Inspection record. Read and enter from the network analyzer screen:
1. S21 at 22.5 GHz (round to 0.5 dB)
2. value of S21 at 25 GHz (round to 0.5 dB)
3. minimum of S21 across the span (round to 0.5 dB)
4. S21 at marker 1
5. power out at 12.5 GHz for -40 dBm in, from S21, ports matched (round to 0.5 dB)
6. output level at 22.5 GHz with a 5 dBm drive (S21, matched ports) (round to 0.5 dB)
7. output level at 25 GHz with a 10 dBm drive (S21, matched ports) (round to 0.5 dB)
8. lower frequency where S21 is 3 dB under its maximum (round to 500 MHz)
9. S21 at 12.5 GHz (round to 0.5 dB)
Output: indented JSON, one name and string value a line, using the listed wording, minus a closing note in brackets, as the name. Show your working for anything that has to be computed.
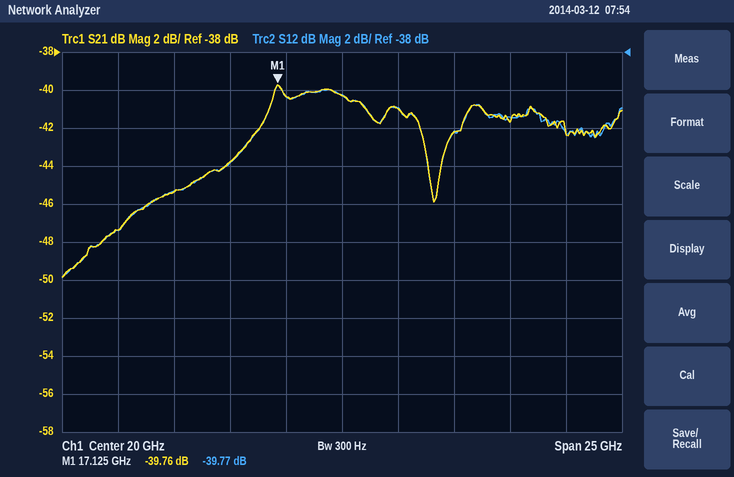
{
  "S21 at 22.5 GHz": "-41.0 dB",
  "value of S21 at 25 GHz": "-42.0 dB",
  "minimum of S21 across the span": "-50.0 dB",
  "S21 at marker 1": "-39.76 dB",
  "power out at 12.5 GHz for -40 dBm in, from S21, ports matched": "-40 dBm + (-45.5 dB) = -85.5 dBm",
  "output level at 22.5 GHz with a 5 dBm drive (S21, matched ports)": "5 dBm + (-41.0 dB) = -36.0 dBm",
  "output level at 25 GHz with a 10 dBm drive (S21, matched ports)": "10 dBm + (-42.0 dB) = -32.0 dBm",
  "lower frequency where S21 is 3 dB under its maximum": "16.0 GHz",
  "S21 at 12.5 GHz": "-45.5 dB"
}
